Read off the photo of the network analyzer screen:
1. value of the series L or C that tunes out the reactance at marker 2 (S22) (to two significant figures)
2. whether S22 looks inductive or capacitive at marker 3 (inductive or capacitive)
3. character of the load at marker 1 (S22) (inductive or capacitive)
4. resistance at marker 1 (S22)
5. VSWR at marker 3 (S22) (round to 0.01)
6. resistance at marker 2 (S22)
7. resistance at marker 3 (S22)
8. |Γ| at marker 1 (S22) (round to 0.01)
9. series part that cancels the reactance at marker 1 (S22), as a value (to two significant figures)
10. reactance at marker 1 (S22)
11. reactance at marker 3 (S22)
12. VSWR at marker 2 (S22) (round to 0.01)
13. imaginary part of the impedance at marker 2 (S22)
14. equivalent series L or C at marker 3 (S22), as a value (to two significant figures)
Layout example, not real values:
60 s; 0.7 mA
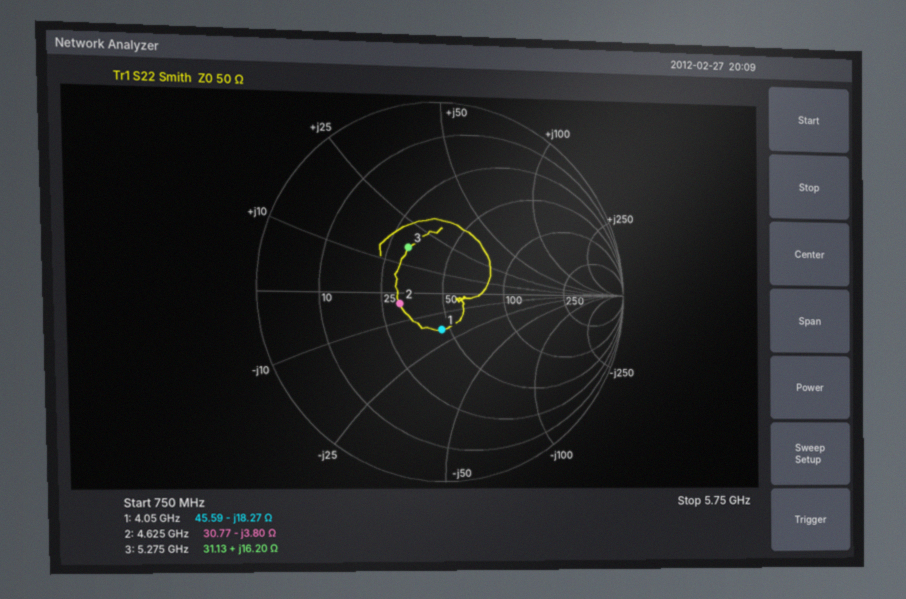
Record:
130 pH; inductive; capacitive; 45.59 Ω; 1.86; 30.77 Ω; 31.13 Ω; 0.19; 720 pH; -18.27 Ω; +16.20 Ω; 1.64; -3.80 Ω; 490 pH
